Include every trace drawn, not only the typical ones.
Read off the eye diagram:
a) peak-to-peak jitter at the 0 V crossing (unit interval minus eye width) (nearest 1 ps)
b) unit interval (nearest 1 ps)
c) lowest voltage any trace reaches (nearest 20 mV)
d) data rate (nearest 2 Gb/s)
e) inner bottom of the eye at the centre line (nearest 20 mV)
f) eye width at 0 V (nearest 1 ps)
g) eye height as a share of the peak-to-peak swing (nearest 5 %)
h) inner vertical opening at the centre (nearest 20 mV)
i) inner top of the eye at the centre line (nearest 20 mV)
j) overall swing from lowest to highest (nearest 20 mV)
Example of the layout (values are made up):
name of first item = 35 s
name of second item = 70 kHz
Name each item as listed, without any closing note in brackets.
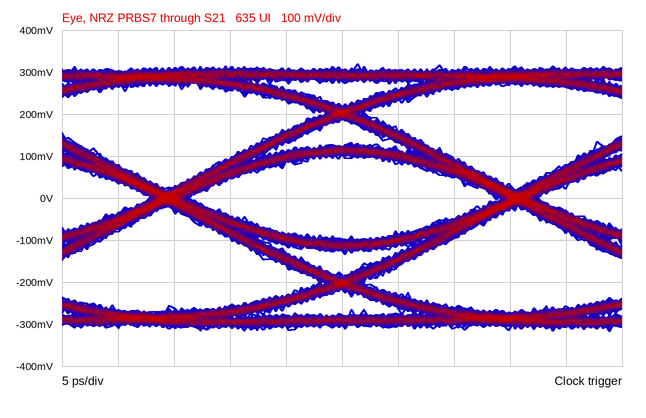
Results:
peak-to-peak jitter at the 0 V crossing (unit interval minus eye width) = 4 ps
unit interval = 31 ps
lowest voltage any trace reaches = -320 mV
data rate = 32 Gb/s
inner bottom of the eye at the centre line = -100 mV
eye width at 0 V = 27 ps
eye height as a share of the peak-to-peak swing = 30 %
inner vertical opening at the centre = 200 mV
inner top of the eye at the centre line = 100 mV
overall swing from lowest to highest = 640 mV
